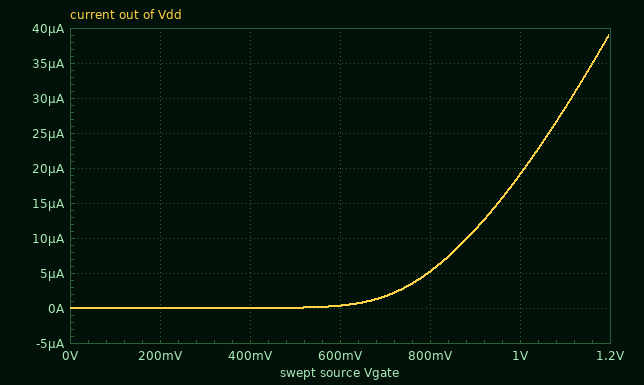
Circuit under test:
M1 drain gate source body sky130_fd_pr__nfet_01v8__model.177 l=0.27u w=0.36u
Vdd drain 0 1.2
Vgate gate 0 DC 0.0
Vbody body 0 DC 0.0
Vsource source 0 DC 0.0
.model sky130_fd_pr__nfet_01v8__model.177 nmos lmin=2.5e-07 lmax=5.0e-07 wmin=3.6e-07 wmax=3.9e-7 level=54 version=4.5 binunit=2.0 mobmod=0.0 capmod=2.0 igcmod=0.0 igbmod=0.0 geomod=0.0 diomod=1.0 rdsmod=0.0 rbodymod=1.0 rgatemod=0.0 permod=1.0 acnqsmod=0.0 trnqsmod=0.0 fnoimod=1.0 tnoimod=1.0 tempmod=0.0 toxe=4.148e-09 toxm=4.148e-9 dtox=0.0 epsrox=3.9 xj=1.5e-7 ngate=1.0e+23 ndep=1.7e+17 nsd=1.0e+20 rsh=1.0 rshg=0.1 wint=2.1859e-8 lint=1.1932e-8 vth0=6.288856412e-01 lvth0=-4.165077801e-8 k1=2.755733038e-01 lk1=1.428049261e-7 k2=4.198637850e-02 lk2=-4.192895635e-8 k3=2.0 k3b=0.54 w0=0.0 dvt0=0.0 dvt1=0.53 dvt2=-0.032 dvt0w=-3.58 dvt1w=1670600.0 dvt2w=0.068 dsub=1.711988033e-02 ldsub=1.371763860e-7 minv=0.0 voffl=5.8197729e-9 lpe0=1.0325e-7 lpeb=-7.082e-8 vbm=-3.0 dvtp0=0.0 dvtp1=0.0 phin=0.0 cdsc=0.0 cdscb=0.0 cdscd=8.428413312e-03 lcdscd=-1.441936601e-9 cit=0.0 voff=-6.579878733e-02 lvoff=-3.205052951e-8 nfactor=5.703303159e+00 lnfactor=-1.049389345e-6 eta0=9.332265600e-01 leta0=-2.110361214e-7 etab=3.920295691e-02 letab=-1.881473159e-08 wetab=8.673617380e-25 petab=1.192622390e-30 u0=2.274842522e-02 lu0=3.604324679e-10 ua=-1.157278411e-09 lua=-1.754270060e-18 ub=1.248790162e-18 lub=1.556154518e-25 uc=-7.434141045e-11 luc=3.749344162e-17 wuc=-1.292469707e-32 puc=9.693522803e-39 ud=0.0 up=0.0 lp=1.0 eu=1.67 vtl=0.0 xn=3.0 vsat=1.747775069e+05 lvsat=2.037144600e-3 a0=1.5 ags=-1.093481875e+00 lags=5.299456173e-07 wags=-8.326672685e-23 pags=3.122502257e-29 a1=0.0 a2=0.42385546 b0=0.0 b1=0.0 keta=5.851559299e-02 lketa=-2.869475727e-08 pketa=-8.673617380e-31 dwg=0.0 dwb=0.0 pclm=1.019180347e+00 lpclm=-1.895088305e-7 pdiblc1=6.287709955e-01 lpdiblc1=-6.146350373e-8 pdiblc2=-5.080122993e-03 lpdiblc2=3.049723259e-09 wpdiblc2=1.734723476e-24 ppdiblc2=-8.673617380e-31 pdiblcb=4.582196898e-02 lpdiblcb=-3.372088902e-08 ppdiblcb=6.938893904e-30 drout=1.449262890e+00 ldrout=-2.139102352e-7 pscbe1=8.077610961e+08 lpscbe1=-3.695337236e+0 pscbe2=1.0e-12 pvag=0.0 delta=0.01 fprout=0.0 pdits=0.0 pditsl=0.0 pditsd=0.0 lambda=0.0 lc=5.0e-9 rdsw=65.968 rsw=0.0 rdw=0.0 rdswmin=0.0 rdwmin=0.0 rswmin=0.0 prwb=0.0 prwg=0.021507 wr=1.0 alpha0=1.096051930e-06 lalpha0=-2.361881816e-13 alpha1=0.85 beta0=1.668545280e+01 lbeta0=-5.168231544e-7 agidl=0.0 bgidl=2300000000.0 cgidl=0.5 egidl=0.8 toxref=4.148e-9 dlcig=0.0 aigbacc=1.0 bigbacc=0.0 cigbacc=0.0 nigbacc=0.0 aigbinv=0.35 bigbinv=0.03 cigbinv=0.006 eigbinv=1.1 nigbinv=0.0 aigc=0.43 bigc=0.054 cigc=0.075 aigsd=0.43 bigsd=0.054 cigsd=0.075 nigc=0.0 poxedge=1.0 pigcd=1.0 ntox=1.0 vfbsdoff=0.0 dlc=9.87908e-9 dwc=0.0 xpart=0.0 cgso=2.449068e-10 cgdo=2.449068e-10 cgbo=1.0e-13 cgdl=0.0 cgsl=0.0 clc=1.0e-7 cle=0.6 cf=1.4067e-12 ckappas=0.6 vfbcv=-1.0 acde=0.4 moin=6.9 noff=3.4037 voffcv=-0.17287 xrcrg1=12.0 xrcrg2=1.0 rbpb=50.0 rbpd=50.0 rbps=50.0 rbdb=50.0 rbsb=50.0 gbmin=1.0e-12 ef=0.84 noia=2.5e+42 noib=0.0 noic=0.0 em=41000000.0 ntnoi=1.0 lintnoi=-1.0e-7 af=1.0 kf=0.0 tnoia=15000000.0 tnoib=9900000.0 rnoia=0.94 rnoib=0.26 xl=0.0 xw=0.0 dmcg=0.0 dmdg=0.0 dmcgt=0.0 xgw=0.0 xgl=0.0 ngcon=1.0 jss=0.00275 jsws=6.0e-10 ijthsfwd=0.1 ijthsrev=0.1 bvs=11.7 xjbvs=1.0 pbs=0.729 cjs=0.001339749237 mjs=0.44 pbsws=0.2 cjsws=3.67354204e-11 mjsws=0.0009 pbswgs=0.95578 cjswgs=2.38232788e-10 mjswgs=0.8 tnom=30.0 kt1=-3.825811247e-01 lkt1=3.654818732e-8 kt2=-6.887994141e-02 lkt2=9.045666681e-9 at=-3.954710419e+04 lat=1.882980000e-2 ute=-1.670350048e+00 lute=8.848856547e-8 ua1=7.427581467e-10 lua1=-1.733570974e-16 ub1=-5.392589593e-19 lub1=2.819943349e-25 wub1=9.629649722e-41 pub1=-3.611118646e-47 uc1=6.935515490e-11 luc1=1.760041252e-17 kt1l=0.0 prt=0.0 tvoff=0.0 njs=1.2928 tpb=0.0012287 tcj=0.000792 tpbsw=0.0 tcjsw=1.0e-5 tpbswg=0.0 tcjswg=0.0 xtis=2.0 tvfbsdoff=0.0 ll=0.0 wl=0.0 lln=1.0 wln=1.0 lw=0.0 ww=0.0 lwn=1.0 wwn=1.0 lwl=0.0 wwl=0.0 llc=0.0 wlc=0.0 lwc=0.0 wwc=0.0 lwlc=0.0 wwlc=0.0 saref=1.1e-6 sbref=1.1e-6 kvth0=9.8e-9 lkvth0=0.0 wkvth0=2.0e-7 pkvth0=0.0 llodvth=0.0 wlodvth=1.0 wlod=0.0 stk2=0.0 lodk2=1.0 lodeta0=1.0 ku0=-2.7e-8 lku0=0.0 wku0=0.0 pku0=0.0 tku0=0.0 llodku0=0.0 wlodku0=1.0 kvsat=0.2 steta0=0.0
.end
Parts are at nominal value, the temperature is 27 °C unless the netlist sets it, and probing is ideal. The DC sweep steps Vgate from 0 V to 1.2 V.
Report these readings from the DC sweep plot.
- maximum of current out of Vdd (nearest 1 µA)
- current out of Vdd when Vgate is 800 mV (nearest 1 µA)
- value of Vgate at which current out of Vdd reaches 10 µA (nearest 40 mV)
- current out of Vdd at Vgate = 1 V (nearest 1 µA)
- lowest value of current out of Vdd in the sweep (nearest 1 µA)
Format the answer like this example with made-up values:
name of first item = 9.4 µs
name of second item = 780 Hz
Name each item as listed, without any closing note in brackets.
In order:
maximum of current out of Vdd = 39 µA
current out of Vdd when Vgate is 800 mV = 5 µA
value of Vgate at which current out of Vdd reaches 10 µA = 880 mV
current out of Vdd at Vgate = 1 V = 19 µA
lowest value of current out of Vdd in the sweep = 0 A
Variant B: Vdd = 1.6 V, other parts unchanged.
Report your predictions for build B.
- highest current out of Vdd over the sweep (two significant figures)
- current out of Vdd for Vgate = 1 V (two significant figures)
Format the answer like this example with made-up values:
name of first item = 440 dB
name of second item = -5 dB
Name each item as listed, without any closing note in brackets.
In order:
highest current out of Vdd over the sweep = 40 µA
current out of Vdd for Vgate = 1 V = 20 µA
